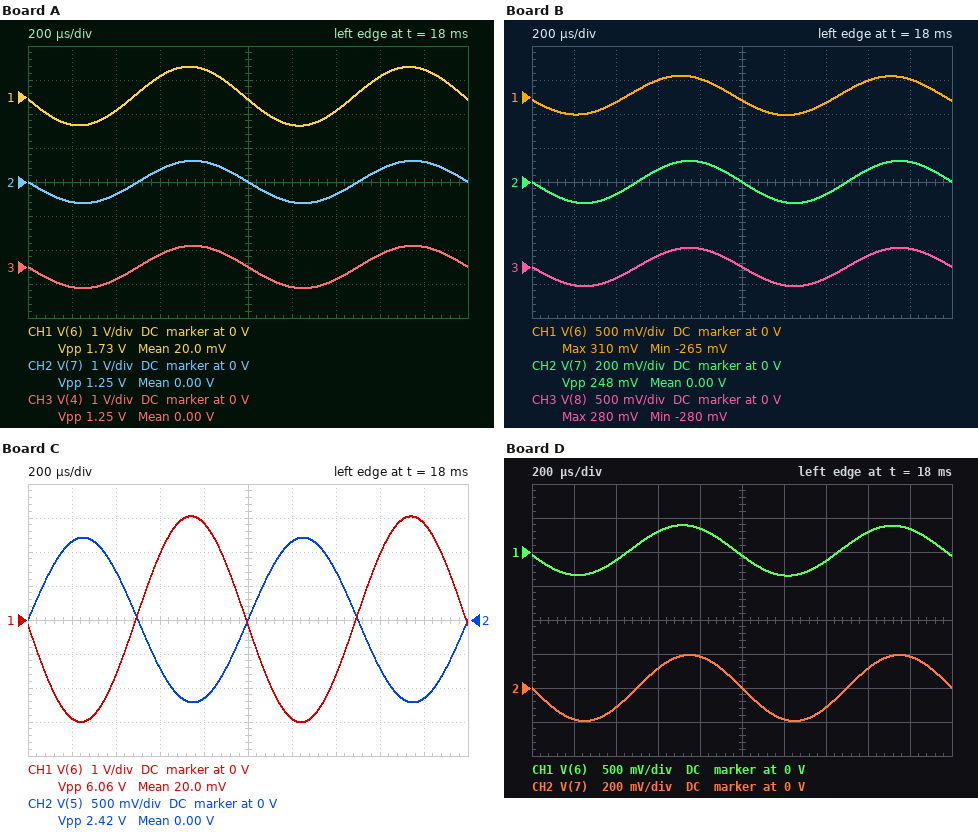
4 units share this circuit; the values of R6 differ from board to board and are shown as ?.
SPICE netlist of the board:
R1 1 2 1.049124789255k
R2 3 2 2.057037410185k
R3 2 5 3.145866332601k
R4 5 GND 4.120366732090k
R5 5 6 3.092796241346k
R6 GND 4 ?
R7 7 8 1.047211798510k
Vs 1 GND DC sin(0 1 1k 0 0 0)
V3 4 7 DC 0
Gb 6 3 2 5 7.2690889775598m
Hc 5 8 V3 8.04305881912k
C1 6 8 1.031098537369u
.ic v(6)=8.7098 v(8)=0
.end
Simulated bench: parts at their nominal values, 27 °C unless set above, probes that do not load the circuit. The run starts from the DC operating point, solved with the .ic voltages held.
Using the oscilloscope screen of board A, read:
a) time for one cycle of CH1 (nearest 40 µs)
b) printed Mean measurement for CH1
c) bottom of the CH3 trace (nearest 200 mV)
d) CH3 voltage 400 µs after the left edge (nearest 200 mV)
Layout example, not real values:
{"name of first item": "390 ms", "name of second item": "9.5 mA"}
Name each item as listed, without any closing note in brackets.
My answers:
{"time for one cycle of CH1": "1.00 ms", "printed Mean measurement for CH1": "20.0 mV", "bottom of the CH3 trace": "-600 mV", "CH3 voltage 400 µs after the left edge": "-400 mV"}
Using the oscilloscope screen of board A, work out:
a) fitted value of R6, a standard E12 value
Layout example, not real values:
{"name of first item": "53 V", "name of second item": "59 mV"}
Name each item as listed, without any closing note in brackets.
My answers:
{"fitted value of R6, a standard E12 value": "2.7 kΩ"}
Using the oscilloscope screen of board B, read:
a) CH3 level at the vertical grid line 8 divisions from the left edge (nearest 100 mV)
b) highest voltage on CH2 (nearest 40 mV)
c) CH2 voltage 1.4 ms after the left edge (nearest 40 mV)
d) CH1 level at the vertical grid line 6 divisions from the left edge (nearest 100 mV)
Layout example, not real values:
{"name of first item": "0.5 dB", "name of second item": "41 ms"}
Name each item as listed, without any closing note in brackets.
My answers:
{"CH3 level at the vertical grid line 8 divisions from the left edge": "200 mV", "highest voltage on CH2": "120 mV", "CH2 voltage 1.4 ms after the left edge": "-80 mV", "CH1 level at the vertical grid line 6 divisions from the left edge": "-300 mV"}
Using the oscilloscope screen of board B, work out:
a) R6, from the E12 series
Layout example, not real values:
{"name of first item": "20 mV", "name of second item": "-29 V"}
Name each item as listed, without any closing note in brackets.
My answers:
{"R6, from the E12 series": "820 Ω"}
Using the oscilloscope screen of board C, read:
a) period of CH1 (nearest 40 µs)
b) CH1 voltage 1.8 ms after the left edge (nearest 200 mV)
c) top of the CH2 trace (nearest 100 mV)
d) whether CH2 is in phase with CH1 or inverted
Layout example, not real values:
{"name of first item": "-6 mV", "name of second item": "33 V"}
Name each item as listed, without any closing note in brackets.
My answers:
{"period of CH1": "1.00 ms", "CH1 voltage 1.8 ms after the left edge": "2.8 V", "top of the CH2 trace": "1.2 V", "whether CH2 is in phase with CH1 or inverted": "inverted"}
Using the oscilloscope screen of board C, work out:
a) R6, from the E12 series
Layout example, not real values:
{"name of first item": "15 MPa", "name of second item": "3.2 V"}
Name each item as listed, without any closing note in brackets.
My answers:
{"R6, from the E12 series": "4.7 kΩ"}
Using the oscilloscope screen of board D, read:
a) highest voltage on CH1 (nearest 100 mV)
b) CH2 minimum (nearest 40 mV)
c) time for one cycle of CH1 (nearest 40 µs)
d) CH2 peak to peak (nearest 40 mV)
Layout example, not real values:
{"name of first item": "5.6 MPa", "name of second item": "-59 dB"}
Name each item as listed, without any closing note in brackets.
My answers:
{"highest voltage on CH1": "400 mV", "CH2 minimum": "-200 mV", "time for one cycle of CH1": "1.00 ms", "CH2 peak to peak": "400 mV"}
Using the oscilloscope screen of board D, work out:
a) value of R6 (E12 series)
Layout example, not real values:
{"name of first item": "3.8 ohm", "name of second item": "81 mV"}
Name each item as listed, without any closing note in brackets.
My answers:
{"value of R6": "1.2 kΩ"}
